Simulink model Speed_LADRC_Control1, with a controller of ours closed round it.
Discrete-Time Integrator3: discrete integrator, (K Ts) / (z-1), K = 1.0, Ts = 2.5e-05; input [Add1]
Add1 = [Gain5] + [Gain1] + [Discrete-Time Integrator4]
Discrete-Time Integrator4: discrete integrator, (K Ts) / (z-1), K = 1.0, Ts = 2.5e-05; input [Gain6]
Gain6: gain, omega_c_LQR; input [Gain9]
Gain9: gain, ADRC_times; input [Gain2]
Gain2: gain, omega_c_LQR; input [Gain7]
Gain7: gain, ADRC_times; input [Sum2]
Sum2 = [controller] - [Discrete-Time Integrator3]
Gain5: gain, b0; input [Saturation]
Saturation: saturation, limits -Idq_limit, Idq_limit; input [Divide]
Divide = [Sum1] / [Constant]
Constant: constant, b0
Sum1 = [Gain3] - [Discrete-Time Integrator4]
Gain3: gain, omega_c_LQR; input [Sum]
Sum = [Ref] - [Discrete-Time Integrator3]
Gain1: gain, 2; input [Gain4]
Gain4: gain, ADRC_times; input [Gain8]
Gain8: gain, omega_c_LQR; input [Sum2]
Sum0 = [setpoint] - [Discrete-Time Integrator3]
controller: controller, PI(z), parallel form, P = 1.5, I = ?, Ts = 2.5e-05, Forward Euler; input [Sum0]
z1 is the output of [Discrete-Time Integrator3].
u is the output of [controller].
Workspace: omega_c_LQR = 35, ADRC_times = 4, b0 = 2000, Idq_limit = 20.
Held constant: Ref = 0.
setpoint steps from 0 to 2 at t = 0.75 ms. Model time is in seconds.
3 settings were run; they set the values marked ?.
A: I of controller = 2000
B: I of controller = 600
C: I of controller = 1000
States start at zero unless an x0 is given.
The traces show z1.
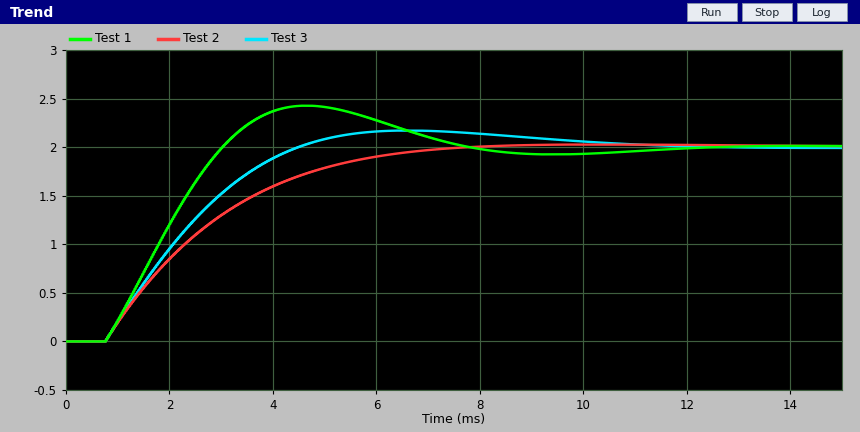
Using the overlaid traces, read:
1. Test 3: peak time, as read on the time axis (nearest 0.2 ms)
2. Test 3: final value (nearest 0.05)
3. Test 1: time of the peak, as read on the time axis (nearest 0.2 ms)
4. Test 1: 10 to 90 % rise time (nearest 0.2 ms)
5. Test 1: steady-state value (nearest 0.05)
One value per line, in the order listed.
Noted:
6.6 ms
2.00
4.6 ms
1.8 ms
2.00
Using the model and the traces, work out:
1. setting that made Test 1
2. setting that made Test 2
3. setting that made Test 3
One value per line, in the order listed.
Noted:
A
B
C
